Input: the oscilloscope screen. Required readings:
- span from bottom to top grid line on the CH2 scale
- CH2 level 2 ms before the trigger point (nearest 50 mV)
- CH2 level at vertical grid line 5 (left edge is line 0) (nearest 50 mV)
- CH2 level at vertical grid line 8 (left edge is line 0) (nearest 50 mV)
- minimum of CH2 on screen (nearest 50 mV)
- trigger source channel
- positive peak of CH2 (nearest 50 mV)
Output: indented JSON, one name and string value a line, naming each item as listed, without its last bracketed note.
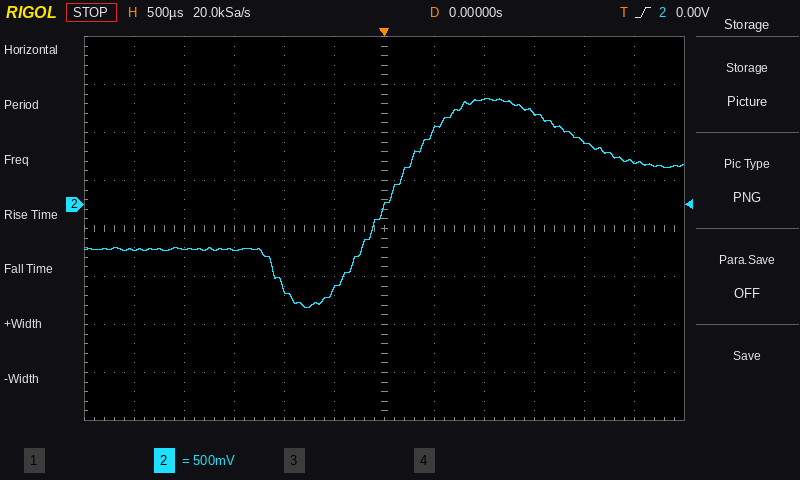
{
  "span from bottom to top grid line on the CH2 scale": "4 V",
  "CH2 level 2 ms before the trigger point": "-450 mV",
  "CH2 level at vertical grid line 5 (left edge is line 0)": "-900 mV",
  "CH2 level at vertical grid line 8 (left edge is line 0)": "1.10 V",
  "minimum of CH2 on screen": "-1.05 V",
  "trigger source channel": "CH2",
  "positive peak of CH2": "1.10 V"
}
